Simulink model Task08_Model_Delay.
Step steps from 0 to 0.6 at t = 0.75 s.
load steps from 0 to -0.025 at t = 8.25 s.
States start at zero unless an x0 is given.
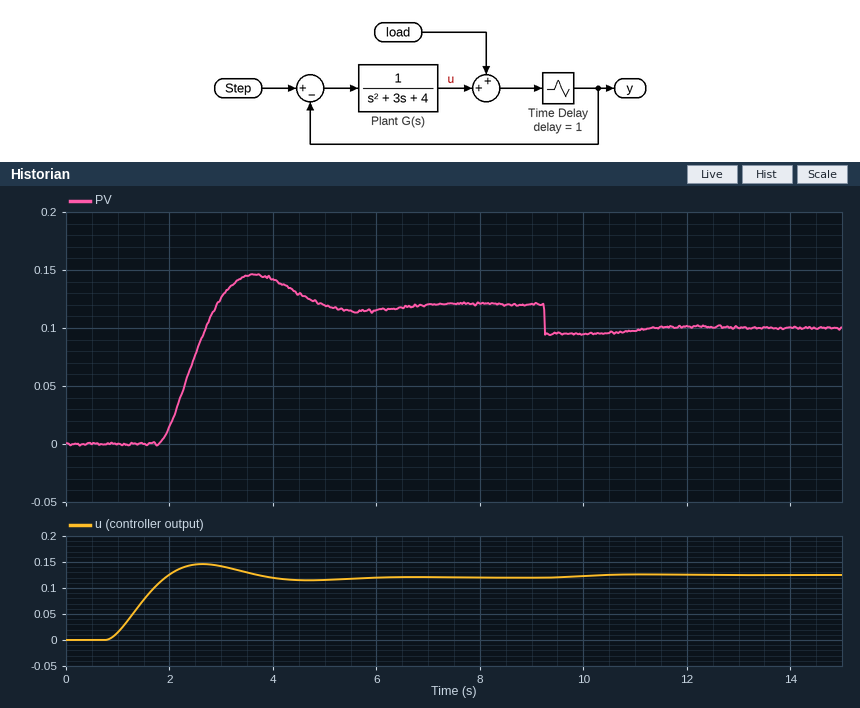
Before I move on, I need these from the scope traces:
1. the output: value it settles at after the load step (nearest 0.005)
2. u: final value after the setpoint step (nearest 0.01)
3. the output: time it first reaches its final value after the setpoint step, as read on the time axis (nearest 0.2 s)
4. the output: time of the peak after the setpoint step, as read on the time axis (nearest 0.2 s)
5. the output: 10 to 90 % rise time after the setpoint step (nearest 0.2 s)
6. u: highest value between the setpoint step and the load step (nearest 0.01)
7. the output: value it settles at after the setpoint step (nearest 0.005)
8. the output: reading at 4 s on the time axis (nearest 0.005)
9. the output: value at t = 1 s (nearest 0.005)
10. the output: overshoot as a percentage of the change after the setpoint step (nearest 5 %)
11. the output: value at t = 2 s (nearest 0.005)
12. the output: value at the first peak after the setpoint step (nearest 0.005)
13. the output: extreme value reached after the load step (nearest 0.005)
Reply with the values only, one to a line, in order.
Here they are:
0.100
0.12
3.0 s
3.6 s
0.8 s
0.15
0.120
0.140
0.000
20 %
0.015
0.145
0.095
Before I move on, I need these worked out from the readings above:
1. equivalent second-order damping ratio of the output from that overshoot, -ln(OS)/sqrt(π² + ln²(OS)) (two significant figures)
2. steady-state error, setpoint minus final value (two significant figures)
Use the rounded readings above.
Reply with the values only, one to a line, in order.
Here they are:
0.46
0.48
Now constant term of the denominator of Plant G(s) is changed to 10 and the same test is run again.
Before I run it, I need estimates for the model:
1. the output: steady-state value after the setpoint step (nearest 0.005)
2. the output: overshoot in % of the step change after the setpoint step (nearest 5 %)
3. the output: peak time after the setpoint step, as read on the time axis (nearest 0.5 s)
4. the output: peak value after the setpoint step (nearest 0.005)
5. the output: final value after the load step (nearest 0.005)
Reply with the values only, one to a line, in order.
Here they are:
0.055
30 %
3.0 s
0.070
0.030
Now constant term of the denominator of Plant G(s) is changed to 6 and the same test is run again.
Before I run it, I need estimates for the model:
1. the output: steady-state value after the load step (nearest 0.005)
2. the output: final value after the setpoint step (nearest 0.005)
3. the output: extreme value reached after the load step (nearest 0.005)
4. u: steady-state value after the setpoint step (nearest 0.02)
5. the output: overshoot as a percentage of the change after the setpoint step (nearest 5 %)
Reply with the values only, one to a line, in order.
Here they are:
0.065
0.085
0.060
0.08
25 %
